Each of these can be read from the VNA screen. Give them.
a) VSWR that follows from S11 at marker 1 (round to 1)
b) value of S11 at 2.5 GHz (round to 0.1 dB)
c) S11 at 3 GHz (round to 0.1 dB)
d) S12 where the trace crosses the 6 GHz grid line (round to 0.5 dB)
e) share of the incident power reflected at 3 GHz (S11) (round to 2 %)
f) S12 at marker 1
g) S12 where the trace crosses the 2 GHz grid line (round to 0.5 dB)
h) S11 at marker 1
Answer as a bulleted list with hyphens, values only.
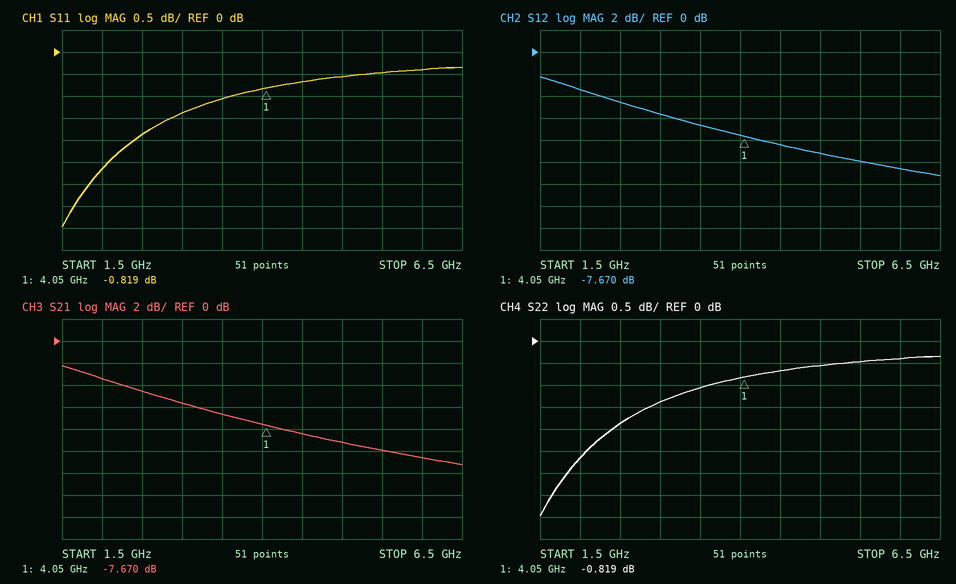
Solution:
- 21
- -1.9 dB
- -1.4 dB
- -10.5 dB
- 72 %
- -7.670 dB
- -3.5 dB
- -0.819 dB
